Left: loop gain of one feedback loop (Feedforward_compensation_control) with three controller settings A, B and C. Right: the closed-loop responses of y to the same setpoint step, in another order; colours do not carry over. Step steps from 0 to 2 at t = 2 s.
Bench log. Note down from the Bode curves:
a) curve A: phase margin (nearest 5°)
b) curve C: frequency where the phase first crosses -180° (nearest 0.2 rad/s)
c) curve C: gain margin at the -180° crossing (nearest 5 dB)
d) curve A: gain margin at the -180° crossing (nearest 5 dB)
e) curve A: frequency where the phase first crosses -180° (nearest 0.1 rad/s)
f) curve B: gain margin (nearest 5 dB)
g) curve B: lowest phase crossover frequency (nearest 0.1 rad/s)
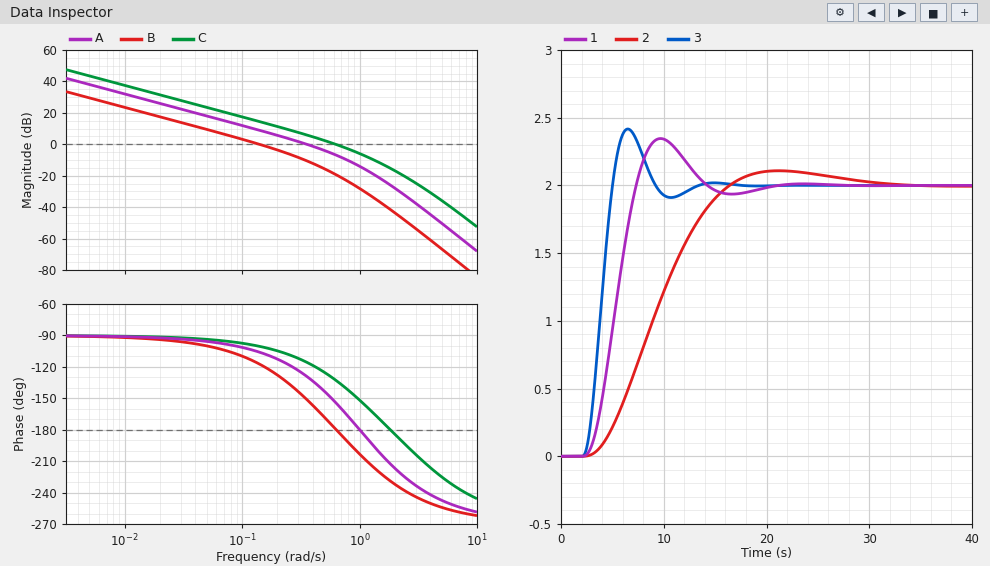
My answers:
50°
1.8 rad/s
15 dB
15 dB
1.0 rad/s
20 dB
0.6 rad/s
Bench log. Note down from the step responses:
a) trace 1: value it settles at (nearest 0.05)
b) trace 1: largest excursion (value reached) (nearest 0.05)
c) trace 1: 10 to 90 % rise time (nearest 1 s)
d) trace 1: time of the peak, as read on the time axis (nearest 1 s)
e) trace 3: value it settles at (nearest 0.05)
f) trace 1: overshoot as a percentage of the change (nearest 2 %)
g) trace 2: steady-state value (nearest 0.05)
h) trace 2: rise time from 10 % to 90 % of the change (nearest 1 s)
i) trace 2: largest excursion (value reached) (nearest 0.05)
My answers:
2.00
2.35
3 s
10 s
2.00
18 %
2.00
9 s
2.10
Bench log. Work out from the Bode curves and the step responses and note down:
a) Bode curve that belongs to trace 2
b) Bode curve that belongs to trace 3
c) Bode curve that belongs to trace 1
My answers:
B
C
A
